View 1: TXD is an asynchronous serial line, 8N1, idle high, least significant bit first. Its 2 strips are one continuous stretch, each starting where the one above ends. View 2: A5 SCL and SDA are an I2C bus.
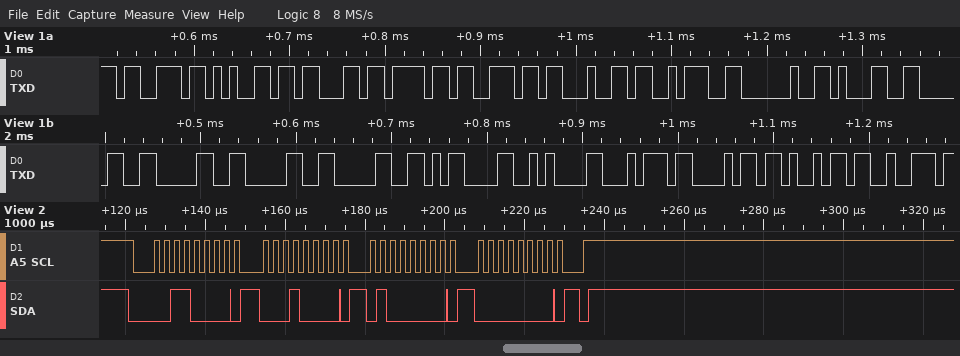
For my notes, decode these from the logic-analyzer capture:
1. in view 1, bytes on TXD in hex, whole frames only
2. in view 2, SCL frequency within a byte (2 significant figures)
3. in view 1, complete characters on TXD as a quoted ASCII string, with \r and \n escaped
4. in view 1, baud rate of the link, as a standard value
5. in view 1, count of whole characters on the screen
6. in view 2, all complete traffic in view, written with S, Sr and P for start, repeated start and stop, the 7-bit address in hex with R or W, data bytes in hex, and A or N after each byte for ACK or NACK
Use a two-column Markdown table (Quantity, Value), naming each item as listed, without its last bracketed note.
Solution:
| Quantity | Value |
|---|---|
| in view 1, bytes on TXD in hex, whole frames only | 0x73 0x65 0x63 0x6F 0x6E 0x64 0x3A 0x20 0x31 0x30 0x30 0x30 0x30 0x0D 0x0A 0x74 0x68 0x69 0x72 |
| in view 2, SCL frequency within a byte | 400 kHz |
| in view 1, complete characters on TXD as a quoted ASCII string, with \r and \n escaped | "second: 10000\r\nthir" |
| in view 1, baud rate of the link, as a standard value | 115200 baud |
| in view 1, count of whole characters on the screen | 19 |
| in view 2, all complete traffic in view, written with S, Sr and P for start, repeated start and stop, the 7-bit address in hex with R or W, data bytes in hex, and A or N after each byte for ACK or NACK | S 18W A 10 A 40 A 00 A P |
